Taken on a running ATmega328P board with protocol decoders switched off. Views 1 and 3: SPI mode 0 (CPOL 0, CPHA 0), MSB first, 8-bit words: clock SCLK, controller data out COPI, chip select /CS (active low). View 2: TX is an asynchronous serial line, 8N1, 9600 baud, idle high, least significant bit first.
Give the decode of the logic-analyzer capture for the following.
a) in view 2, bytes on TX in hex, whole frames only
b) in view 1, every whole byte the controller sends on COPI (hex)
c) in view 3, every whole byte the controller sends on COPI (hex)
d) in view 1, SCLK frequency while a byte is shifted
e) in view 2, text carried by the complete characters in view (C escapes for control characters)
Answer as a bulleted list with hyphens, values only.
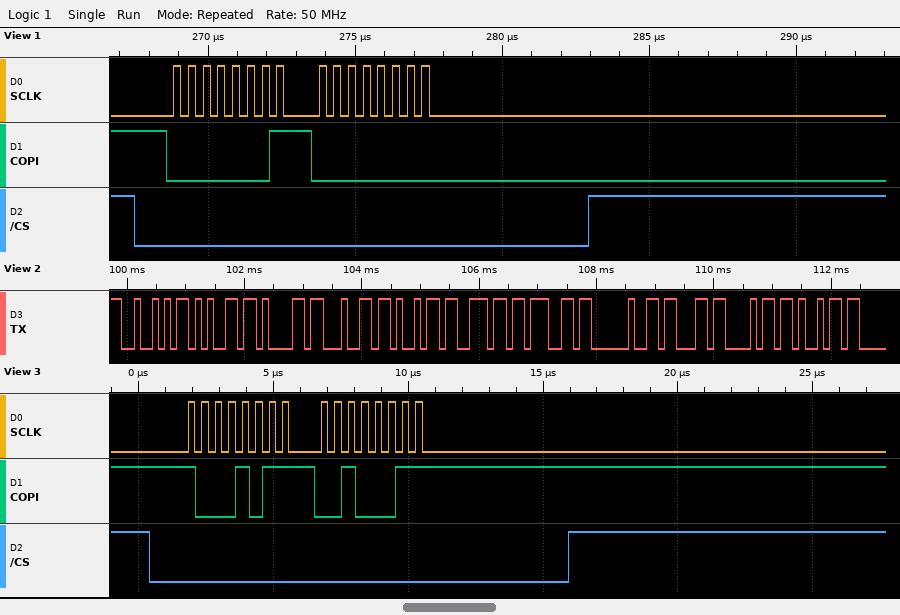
- 0x52 0x65 0x61 0x64 0x69 0x6E 0x67 0x20 0x63 0x68 0x69
- 01 00
- 8B 23
- 2 MHz
- "Reading chi"
